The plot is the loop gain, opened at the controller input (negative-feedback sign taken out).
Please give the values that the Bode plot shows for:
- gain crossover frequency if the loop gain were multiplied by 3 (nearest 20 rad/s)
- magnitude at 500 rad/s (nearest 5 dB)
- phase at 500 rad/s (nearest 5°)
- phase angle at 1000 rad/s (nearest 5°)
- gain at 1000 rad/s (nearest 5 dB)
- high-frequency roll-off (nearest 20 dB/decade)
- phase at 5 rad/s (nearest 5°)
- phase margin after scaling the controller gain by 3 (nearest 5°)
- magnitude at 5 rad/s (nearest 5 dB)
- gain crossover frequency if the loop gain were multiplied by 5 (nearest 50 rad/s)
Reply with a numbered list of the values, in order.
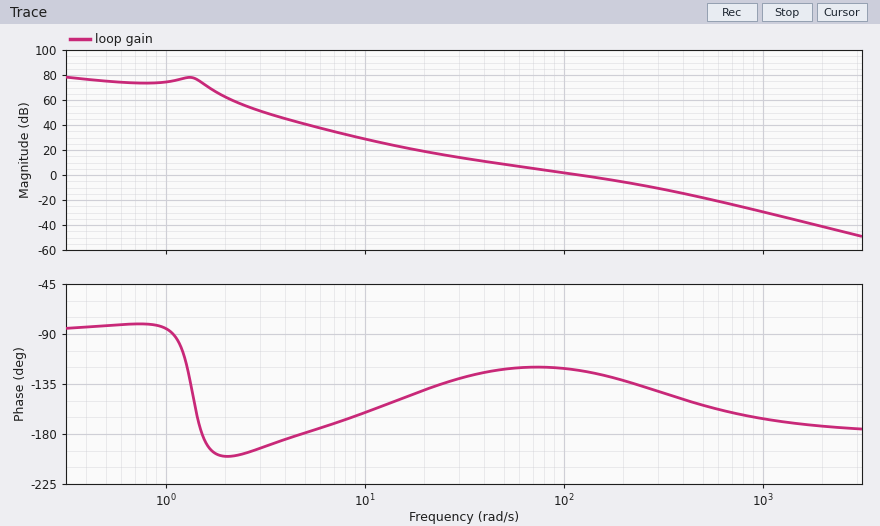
1. 280 rad/s
2. -20 dB
3. -155°
4. -165°
5. -30 dB
6. -40 dB/decade
7. -180°
8. 40°
9. 40 dB
10. 400 rad/s
